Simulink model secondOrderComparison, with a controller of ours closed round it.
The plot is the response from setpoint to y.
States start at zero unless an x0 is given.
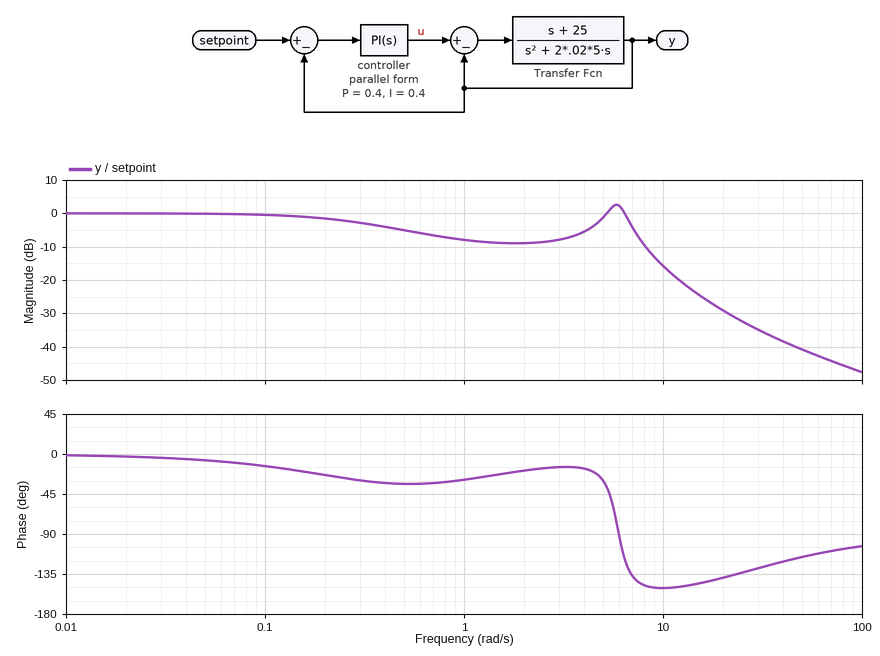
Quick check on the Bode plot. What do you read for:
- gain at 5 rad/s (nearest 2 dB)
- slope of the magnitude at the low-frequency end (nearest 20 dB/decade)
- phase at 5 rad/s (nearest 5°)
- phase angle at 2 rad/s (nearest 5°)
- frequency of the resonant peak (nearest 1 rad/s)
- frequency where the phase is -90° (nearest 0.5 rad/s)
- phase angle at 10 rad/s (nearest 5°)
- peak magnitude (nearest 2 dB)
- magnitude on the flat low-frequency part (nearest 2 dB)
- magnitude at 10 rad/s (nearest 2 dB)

-2 dB
0 dB/decade
-30°
-20°
6 rad/s
6.0 rad/s
-150°
2 dB
0 dB
-16 dB
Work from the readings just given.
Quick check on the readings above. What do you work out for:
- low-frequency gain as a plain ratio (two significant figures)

1.0
